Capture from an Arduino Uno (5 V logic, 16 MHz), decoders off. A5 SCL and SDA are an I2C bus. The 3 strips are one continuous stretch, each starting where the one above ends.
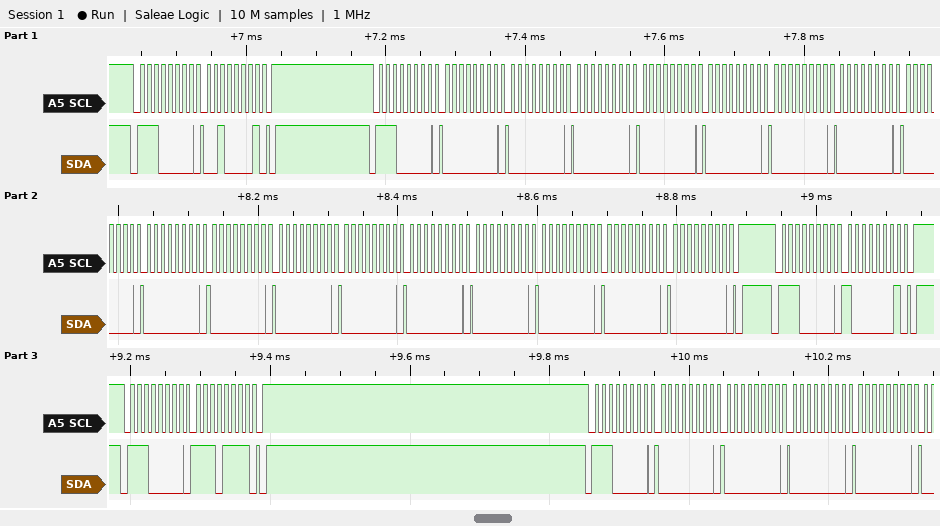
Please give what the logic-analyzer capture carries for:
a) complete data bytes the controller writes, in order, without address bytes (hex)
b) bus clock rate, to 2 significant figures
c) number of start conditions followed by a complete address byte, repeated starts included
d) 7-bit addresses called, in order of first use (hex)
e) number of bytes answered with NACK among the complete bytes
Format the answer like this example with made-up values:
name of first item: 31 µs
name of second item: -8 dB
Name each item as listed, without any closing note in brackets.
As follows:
complete data bytes the controller writes, in order, without address bytes: 21 00 00 00 00 00 00 00 00 00 00 00 00 00 00 00 00 00 81 EF 00 00 00 00
bus clock rate, to 2 significant figures: 100 kHz
number of start conditions followed by a complete address byte, repeated starts included: 5
7-bit addresses called, in order of first use: 0x70
number of bytes answered with NACK among the complete bytes: 0
